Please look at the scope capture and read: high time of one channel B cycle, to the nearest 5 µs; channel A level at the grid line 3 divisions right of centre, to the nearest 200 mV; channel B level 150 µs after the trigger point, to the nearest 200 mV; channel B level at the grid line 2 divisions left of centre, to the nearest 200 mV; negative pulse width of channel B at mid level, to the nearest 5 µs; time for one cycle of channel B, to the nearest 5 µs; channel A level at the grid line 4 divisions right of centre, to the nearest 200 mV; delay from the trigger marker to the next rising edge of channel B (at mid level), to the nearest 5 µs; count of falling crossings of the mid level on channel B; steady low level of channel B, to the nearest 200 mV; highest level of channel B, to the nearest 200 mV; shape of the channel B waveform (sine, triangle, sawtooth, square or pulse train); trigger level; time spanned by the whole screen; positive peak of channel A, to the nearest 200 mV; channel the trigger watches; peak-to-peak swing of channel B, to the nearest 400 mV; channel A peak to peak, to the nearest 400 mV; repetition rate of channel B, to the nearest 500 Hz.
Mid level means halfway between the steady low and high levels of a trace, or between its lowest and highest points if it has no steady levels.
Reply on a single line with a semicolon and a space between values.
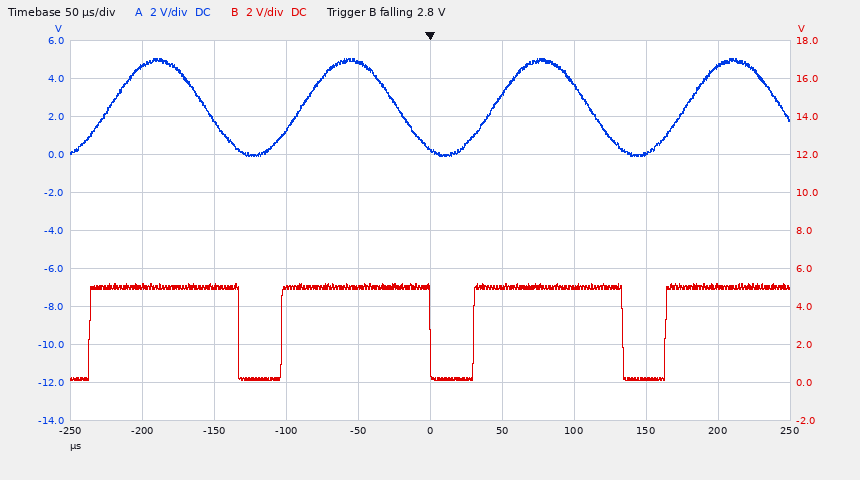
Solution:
105 µs; 0.0 V; 200 mV; 5.0 V; 30 µs; 135 µs; 4.6 V; 30 µs; 3; 200 mV; 5.2 V; pulse train; 2.8 V; 500 µs; 5.0 V; channel B; 5.2 V; 5.2 V; 7.5 kHz
